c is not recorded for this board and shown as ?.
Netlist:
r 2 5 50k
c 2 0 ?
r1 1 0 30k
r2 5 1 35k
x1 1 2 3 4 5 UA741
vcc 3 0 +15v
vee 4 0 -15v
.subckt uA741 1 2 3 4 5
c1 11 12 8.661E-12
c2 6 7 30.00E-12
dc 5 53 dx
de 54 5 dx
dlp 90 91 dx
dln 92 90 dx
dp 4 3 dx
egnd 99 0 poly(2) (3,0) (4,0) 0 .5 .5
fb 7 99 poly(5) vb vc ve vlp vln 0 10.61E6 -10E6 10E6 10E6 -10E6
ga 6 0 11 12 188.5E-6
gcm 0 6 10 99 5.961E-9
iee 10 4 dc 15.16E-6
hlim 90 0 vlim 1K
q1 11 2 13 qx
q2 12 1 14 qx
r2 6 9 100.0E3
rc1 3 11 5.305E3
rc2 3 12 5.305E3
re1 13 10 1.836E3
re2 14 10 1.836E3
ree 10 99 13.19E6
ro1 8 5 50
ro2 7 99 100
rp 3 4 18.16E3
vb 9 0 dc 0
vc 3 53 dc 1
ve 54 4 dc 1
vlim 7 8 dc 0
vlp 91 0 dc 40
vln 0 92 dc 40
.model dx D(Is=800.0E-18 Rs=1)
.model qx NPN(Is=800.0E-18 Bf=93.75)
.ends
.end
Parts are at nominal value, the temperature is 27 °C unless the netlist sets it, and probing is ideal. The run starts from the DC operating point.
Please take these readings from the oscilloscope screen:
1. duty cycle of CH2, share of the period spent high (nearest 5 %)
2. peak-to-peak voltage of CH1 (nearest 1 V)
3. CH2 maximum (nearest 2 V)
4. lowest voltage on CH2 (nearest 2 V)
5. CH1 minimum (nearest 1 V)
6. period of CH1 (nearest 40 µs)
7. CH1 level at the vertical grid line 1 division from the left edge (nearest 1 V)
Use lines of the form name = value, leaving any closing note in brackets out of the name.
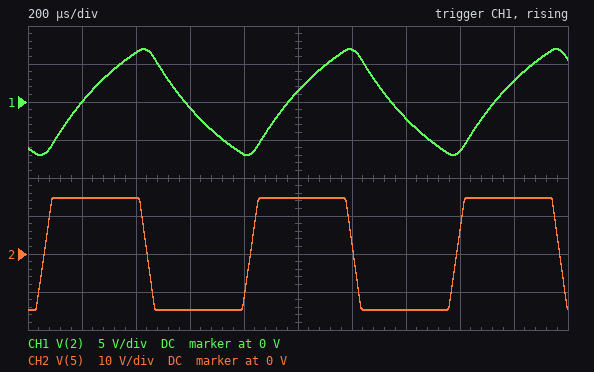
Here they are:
duty cycle of CH2, share of the period spent high = 50 %
peak-to-peak voltage of CH1 = 14 V
CH2 maximum = 14 V
lowest voltage on CH2 = -14 V
CH1 minimum = -7 V
period of CH1 = 760 µs
CH1 level at the vertical grid line 1 division from the left edge = 0 V
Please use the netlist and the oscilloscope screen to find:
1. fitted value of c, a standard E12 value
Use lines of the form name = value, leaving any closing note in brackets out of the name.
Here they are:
fitted value of c, a standard E12 value = 6.8 nF
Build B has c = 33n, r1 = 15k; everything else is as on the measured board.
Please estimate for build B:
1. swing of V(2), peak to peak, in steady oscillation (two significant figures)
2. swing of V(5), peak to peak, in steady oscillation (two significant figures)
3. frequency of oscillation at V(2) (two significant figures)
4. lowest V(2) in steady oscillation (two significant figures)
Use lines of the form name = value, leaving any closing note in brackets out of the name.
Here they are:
swing of V(2), peak to peak, in steady oscillation = 8.9 V
swing of V(5), peak to peak, in steady oscillation = 29 V
frequency of oscillation at V(2) = 470 Hz
lowest V(2) in steady oscillation = -4.5 V
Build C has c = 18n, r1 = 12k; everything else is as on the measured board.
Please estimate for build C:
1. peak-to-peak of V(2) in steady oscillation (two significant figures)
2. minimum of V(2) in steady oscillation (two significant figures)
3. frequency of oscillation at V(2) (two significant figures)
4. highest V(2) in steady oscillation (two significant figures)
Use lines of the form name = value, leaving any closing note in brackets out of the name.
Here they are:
peak-to-peak of V(2) in steady oscillation = 7.8 V
minimum of V(2) in steady oscillation = -3.9 V
frequency of oscillation at V(2) = 960 Hz
highest V(2) in steady oscillation = 3.9 V
